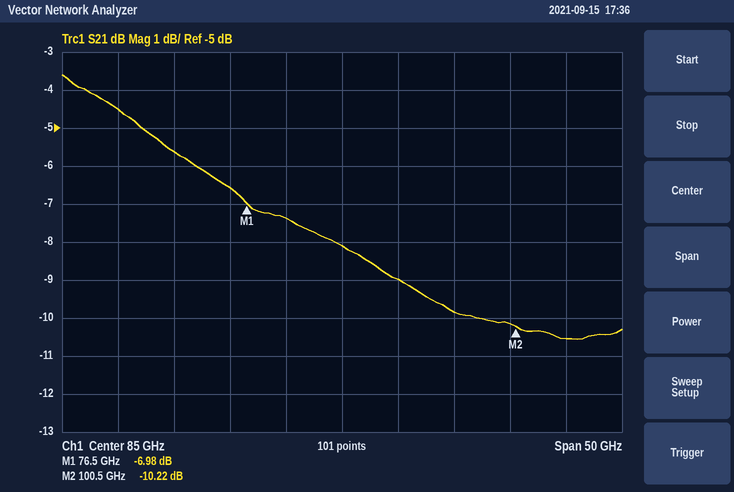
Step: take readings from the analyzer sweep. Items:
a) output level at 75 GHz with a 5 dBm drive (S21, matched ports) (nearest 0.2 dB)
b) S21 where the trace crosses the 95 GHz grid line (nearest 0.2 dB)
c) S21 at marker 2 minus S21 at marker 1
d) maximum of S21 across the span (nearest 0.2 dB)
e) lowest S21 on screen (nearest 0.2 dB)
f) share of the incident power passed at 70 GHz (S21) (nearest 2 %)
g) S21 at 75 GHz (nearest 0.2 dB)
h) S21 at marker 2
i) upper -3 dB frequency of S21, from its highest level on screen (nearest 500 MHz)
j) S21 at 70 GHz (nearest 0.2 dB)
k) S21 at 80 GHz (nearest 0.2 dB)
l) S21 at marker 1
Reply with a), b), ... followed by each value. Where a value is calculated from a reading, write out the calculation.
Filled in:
a) 5 dBm + (-6.6 dB) = -1.6 dBm
b) -9.8 dB
c) -10.22 − (-6.98) = -3.24 dB
d) -3.6 dB
e) -10.6 dB
f) 10^(-5.6/10) ≈ 28 %
g) -6.6 dB
h) -10.22 dB
i) 75.0 GHz
j) -5.6 dB
k) -7.4 dB
l) -6.98 dB
